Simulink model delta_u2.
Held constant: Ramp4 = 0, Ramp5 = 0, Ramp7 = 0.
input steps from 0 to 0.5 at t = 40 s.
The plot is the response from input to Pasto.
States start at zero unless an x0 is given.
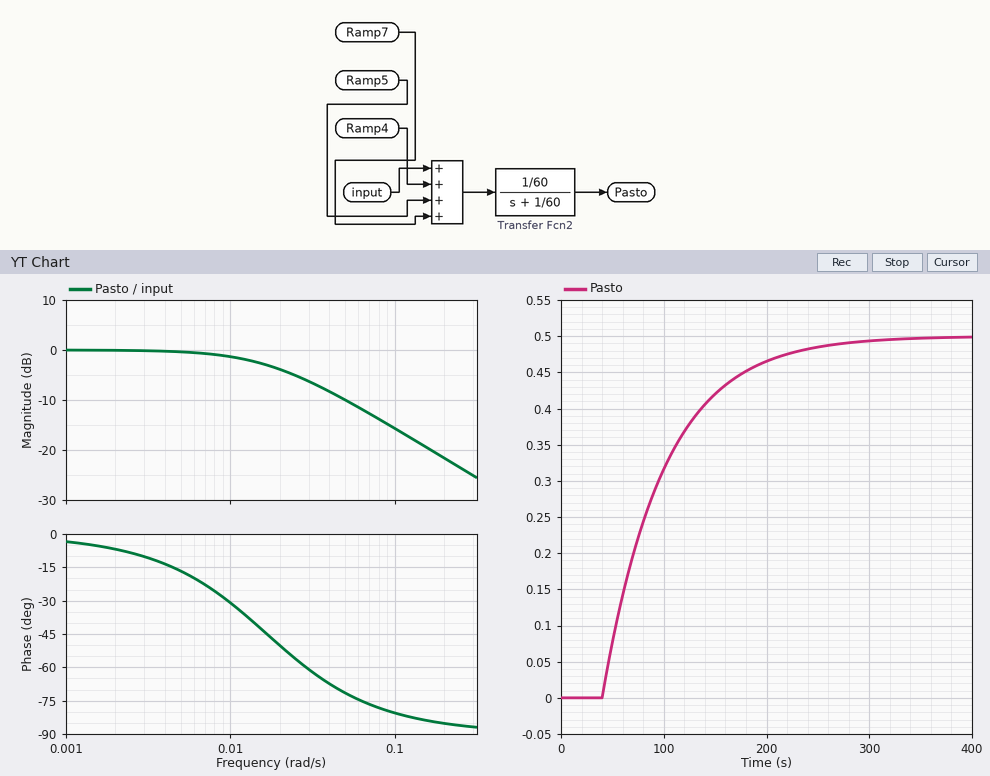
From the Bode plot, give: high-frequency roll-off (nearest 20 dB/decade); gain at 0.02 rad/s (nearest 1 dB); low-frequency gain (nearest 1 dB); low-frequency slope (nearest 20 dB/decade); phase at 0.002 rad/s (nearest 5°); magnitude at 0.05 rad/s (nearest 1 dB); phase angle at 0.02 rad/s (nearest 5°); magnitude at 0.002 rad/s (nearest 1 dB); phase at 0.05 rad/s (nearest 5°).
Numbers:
-20 dB/decade
-4 dB
0 dB
0 dB/decade
-5°
-10 dB
-50°
0 dB
-70°
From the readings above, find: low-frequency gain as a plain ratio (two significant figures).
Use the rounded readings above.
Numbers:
1.0
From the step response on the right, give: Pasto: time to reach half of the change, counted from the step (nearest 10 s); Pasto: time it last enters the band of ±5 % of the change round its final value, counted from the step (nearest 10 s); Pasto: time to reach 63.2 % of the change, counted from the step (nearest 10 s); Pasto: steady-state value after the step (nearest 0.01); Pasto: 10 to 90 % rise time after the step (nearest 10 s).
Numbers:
40 s
180 s
60 s
0.50
130 s
